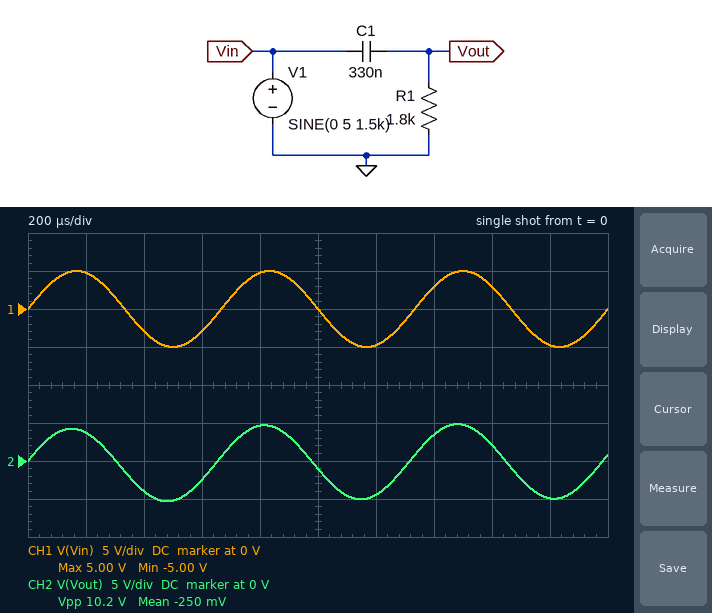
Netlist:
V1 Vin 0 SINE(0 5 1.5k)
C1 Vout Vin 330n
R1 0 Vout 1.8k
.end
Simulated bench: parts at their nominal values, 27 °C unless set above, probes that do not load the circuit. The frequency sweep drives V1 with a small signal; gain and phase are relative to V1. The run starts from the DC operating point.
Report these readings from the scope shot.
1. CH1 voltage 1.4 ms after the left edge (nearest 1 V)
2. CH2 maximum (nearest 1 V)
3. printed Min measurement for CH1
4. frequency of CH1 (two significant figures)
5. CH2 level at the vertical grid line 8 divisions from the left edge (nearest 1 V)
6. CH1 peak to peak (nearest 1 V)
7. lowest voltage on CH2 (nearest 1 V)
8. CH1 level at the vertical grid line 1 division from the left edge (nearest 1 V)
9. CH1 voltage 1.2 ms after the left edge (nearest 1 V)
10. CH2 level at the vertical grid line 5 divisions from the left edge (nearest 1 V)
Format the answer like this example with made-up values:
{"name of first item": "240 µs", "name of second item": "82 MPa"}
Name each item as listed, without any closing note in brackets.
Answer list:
{"CH1 voltage 1.4 ms after the left edge": "3 V", "CH2 maximum": "5 V", "printed Min measurement for CH1": "-5.00 V", "frequency of CH1": "1.5 kHz", "CH2 level at the vertical grid line 8 divisions from the left edge": "2 V", "CH1 peak to peak": "10 V", "lowest voltage on CH2": "-5 V", "CH1 level at the vertical grid line 1 division from the left edge": "5 V", "CH1 voltage 1.2 ms after the left edge": "-5 V", "CH2 level at the vertical grid line 5 divisions from the left edge": "-1 V"}
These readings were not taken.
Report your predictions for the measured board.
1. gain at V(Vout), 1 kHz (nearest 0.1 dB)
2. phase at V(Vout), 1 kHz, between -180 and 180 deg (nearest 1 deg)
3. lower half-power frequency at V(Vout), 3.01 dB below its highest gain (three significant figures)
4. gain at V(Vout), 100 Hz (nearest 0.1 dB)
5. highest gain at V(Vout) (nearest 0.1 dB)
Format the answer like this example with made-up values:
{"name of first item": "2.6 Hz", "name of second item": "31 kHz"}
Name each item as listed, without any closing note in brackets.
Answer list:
{"gain at V(Vout), 1 kHz": "-0.3 dB", "phase at V(Vout), 1 kHz, between -180 and 180 deg": "15 deg", "lower half-power frequency at V(Vout), 3.01 dB below its highest gain": "268 Hz", "gain at V(Vout), 100 Hz": "-9.1 dB", "highest gain at V(Vout)": "0 dB"}
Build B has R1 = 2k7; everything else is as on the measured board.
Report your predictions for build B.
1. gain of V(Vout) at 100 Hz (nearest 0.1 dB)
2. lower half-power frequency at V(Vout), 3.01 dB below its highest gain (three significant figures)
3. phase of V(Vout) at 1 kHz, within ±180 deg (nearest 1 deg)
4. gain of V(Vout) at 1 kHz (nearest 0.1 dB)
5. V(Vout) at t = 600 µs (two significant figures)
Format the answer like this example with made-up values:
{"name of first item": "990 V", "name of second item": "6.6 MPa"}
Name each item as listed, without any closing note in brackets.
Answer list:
{"gain of V(Vout) at 100 Hz": "-6.2 dB", "lower half-power frequency at V(Vout), 3.01 dB below its highest gain": "179 Hz", "phase of V(Vout) at 1 kHz, within ±180 deg": "10 deg", "gain of V(Vout) at 1 kHz": "-0.1 dB", "V(Vout) at t = 600 µs": "-2.7 V"}
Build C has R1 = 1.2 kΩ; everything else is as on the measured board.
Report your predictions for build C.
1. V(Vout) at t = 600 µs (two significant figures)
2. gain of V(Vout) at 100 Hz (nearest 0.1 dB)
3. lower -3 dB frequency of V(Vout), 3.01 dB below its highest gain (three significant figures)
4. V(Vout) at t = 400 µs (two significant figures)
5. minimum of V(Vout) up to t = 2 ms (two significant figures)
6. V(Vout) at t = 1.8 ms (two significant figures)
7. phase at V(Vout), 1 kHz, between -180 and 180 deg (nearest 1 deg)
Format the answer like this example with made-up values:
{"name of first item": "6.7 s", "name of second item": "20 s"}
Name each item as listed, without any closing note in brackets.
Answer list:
{"V(Vout) at t = 600 µs": "-2.0 V", "gain of V(Vout) at 100 Hz": "-12.3 dB", "lower -3 dB frequency of V(Vout), 3.01 dB below its highest gain": "402 Hz", "V(Vout) at t = 400 µs": "-4.2 V", "minimum of V(Vout) up to t = 2 ms": "-5.2 V", "V(Vout) at t = 1.8 ms": "-4.8 V", "phase at V(Vout), 1 kHz, between -180 and 180 deg": "22 deg"}
